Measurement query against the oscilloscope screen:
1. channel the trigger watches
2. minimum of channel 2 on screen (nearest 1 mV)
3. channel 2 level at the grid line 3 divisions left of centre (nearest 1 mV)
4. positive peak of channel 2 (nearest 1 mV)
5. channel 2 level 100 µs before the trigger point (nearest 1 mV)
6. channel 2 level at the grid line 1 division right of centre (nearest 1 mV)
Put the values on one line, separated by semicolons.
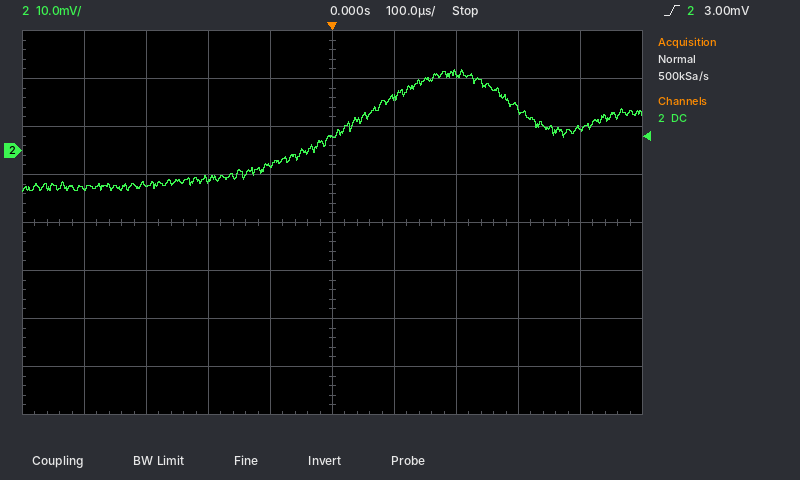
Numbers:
channel 2; -9 mV; -7 mV; 17 mV; -3 mV; 11 mV
